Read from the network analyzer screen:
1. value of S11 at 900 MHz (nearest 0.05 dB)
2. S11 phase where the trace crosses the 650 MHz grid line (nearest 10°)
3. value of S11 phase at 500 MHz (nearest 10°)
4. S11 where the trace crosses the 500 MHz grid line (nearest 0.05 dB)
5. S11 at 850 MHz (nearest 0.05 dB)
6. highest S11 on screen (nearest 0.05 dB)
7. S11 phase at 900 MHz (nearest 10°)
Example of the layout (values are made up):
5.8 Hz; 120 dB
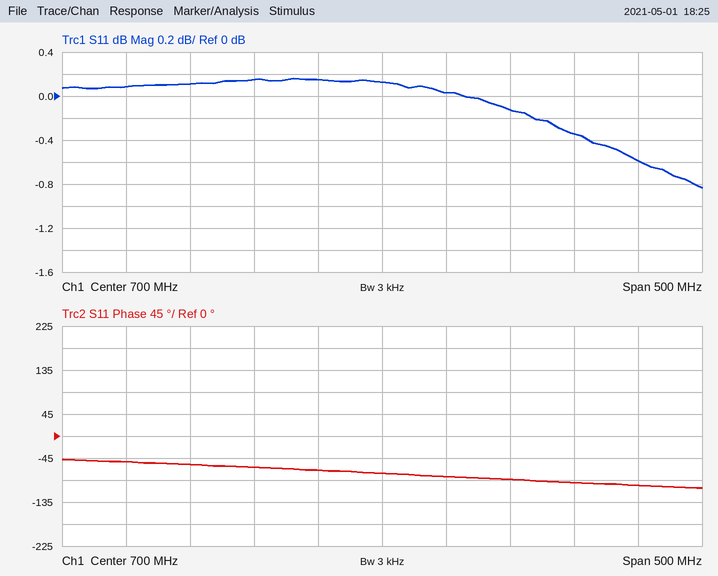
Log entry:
-0.60 dB; -70°; -50°; 0.10 dB; -0.35 dB; 0.15 dB; -100°
